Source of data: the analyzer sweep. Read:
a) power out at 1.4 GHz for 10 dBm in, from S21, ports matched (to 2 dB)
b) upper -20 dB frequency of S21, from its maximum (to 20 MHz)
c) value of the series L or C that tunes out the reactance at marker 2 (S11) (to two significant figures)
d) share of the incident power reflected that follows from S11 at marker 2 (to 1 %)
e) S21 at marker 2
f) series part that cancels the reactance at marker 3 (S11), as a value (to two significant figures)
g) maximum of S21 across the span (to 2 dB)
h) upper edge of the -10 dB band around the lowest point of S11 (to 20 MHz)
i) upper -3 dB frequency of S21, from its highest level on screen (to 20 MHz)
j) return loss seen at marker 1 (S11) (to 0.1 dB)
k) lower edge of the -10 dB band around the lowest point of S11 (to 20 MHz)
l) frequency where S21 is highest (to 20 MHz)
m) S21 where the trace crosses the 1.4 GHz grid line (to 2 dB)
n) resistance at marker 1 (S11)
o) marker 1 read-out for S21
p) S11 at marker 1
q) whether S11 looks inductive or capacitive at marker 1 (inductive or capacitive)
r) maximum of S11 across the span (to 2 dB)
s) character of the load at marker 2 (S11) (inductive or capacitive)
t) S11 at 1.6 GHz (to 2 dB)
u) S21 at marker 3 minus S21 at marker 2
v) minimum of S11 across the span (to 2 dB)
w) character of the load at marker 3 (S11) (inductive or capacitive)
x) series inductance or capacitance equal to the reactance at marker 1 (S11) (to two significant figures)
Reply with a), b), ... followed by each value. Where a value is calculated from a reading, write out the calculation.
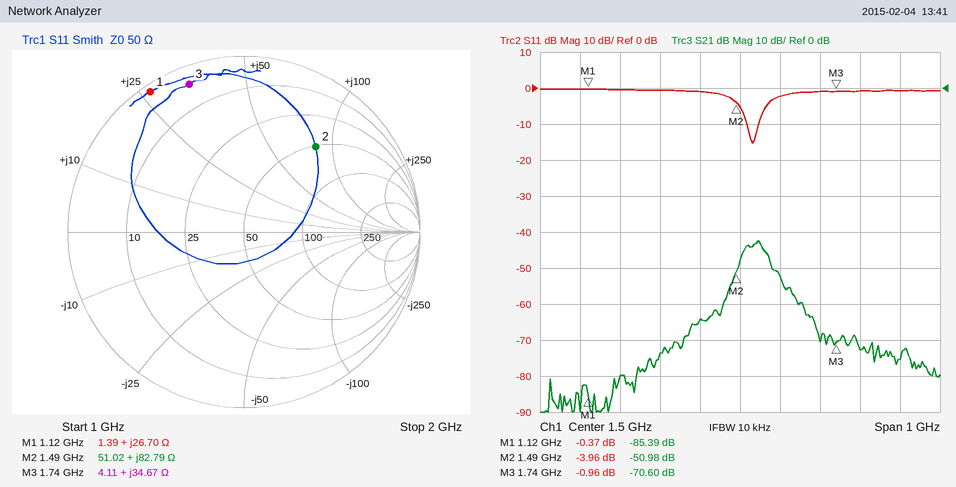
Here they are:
a) 10 dBm + (-64 dB) = -54 dBm
b) 1.66 GHz
c) C = 1/(2π × 1.49 GHz × 82.79 Ω) ≈ 1.3 pF
d) 10^(-3.96/10) ≈ 40 %
e) -50.98 dB
f) C = 1/(2π × 1.74 GHz × 34.67 Ω) ≈ 2.6 pF
g) -42 dB
h) 1.54 GHz
i) 1.56 GHz
j) 0.4 dB
k) 1.52 GHz
l) 1.54 GHz
m) -64 dB
n) 1.39 Ω
o) -85.39 dB
p) -0.37 dB
q) inductive
r) 0 dB
s) inductive
t) -2 dB
u) -70.6 − (-50.98) = -19.62 dB
v) -16 dB
w) inductive
x) L = 26.7 Ω/(2π × 1.12 GHz) ≈ 3.8 nH
